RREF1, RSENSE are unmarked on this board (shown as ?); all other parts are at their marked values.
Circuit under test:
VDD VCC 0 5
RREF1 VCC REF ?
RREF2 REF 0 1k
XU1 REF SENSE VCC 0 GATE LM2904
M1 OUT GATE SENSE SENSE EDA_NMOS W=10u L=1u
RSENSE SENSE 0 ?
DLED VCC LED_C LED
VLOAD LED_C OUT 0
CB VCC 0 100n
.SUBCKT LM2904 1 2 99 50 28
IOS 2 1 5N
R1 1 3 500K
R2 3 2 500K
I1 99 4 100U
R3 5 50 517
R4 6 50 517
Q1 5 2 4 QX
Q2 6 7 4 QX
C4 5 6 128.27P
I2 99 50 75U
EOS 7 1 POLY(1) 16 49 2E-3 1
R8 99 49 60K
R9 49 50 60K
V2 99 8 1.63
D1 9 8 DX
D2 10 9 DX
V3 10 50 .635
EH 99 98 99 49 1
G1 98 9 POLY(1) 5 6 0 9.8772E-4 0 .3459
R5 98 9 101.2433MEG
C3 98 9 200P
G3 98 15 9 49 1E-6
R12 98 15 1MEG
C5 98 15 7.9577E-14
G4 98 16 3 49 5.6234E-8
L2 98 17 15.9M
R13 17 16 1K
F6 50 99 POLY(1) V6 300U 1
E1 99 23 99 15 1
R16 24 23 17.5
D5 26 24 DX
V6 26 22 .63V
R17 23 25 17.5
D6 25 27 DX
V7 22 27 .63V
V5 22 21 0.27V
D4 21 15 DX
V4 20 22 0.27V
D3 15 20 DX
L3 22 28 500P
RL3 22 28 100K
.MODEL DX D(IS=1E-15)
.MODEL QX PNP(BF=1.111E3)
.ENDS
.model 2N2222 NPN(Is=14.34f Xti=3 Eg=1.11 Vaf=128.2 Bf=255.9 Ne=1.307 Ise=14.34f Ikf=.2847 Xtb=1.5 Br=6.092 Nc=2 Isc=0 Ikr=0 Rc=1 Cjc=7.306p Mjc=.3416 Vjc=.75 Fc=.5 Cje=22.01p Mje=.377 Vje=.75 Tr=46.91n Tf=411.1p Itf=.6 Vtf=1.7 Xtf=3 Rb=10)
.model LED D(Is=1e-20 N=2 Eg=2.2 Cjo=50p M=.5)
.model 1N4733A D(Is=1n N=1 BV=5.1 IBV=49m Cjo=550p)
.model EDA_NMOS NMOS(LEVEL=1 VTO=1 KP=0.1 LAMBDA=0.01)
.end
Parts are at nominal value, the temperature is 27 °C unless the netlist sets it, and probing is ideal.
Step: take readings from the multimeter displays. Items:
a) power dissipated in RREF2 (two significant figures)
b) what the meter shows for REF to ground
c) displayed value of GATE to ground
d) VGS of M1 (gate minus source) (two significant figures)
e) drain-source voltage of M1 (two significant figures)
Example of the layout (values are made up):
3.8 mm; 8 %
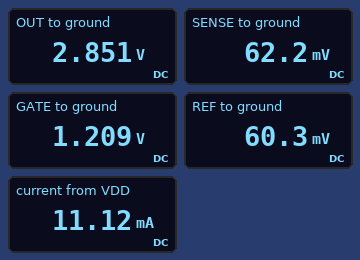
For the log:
3.6 µW; 60.3 mV; 1.209 V; 1.1 V; 2.8 V
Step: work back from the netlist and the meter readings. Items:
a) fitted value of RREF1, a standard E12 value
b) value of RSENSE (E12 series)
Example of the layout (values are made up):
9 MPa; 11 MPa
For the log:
82 kΩ; 5.6 Ω
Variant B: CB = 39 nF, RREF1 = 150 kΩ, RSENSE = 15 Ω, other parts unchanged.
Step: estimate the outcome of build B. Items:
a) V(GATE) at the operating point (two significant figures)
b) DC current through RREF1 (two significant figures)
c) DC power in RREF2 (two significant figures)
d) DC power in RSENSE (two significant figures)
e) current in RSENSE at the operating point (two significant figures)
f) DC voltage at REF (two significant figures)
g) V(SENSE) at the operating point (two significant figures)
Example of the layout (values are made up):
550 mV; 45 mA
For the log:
1.1 V; 33 µA; 1.1 µW; 82 µW; 2.3 mA; 33 mV; 35 mV
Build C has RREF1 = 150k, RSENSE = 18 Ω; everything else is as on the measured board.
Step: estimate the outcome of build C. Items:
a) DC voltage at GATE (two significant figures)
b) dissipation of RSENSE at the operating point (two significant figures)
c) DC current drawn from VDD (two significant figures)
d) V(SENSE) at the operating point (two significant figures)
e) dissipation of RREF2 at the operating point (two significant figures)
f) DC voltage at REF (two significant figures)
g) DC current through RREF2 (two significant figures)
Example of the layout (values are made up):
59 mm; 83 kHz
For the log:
1.1 V; 68 µW; 1.9 mA; 35 mV; 1.1 µW; 33 mV; 33 µA
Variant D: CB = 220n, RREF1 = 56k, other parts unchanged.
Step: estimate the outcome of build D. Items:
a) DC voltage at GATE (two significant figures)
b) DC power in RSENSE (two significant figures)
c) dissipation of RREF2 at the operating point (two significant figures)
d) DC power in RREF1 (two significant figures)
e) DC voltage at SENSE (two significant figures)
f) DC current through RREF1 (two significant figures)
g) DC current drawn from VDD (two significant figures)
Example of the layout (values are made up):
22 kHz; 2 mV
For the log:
1.3 V; 1.4 mW; 7.7 µW; 430 µW; 90 mV; 88 µA; 16 mA
